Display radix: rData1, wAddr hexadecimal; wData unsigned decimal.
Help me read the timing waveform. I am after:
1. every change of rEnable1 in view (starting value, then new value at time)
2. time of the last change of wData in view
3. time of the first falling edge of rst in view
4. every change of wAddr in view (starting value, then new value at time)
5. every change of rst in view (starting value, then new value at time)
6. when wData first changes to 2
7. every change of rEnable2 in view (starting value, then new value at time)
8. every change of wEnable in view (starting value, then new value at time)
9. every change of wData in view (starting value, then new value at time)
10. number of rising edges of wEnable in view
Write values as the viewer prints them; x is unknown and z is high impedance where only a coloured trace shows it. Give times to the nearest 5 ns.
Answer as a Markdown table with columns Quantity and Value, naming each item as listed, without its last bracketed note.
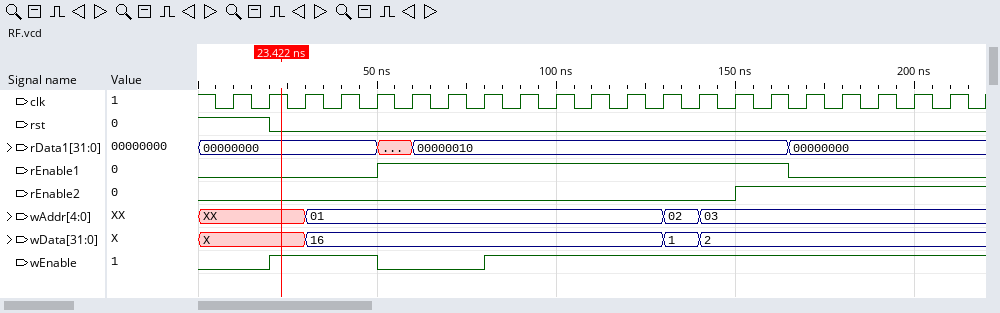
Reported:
| Quantity | Value |
|---|---|
| every change of rEnable1 in view | 0, 1 at 50 ns, 0 at 165 ns |
| time of the last change of wData in view | 140 ns |
| time of the first falling edge of rst in view | 20 ns |
| every change of wAddr in view | XX, 01 at 30 ns, 02 at 130 ns, 03 at 140 ns |
| every change of rst in view | 1, 0 at 20 ns |
| when wData first changes to 2 | 140 ns |
| every change of rEnable2 in view | 0, 1 at 150 ns |
| every change of wEnable in view | 0, 1 at 20 ns, 0 at 50 ns, 1 at 80 ns |
| every change of wData in view | X, 16 at 30 ns, 1 at 130 ns, 2 at 140 ns |
| number of rising edges of wEnable in view | 2 |
